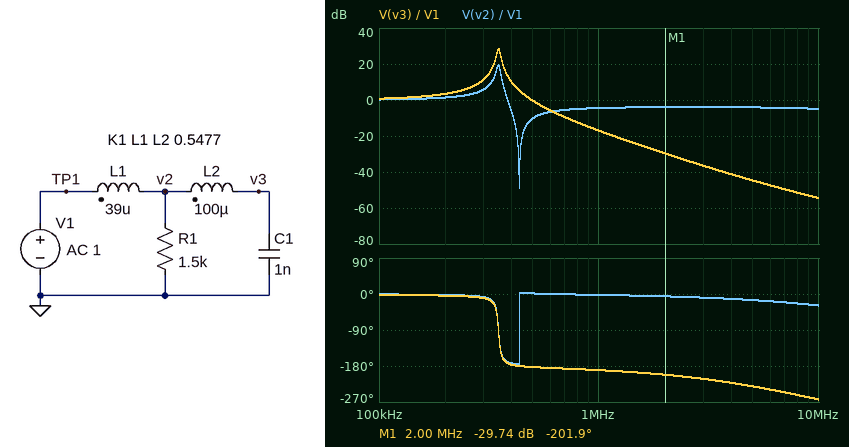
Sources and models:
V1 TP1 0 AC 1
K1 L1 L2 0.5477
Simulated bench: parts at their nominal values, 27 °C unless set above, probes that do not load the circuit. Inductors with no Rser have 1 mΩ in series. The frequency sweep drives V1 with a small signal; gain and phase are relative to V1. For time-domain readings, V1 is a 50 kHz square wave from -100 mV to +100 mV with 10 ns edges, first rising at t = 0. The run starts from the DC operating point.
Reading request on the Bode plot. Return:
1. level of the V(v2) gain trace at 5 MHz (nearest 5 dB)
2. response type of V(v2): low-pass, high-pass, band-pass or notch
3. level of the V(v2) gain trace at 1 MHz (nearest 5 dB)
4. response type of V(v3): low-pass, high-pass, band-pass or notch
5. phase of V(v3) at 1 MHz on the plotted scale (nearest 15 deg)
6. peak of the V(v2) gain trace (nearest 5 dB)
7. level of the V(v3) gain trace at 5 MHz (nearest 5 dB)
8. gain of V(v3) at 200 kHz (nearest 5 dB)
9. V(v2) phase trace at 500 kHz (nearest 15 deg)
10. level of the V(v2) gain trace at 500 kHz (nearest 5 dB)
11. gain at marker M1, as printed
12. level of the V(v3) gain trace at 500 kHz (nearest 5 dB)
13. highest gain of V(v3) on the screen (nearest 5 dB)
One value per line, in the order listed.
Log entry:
-5 dB
band-pass
-5 dB
low-pass
-195 deg
20 dB
-45 dB
5 dB
0 deg
-10 dB
-29.74 dB
0 dB
30 dB
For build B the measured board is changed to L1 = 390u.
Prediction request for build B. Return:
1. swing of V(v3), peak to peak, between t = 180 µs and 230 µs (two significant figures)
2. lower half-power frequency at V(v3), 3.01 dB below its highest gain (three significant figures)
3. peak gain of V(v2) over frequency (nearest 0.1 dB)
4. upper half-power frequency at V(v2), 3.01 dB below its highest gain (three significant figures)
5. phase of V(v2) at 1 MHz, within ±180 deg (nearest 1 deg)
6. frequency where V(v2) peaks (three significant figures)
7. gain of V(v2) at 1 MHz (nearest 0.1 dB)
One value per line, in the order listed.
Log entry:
430 mV
157 kHz
8.3 dB
207 kHz
-6 deg
183 kHz
-11.5 dB
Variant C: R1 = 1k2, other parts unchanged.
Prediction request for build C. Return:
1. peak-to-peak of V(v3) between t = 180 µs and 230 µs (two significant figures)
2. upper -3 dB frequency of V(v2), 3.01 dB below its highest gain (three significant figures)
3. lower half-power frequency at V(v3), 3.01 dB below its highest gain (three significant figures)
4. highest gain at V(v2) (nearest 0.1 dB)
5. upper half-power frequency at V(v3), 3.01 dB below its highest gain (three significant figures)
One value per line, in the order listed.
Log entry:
1.1 V
356 kHz
341 kHz
17.5 dB
358 kHz
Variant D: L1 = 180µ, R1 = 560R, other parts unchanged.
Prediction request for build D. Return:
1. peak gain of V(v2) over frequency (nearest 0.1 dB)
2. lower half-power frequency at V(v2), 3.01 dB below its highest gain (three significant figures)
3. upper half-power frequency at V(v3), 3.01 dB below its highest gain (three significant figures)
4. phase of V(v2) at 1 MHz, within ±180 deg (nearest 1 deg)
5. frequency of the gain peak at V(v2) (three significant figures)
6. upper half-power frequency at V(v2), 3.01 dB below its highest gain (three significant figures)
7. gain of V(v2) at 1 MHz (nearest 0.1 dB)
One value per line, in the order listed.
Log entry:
3.9 dB
108 kHz
285 kHz
-13 deg
222 kHz
265 kHz
-8.9 dB
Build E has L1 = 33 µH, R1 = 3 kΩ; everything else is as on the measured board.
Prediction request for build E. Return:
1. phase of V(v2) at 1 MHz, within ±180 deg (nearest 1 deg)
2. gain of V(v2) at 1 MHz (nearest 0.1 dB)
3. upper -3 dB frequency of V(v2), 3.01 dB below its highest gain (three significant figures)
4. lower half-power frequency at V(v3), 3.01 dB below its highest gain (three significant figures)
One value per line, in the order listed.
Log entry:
-1 deg
-4.1 dB
362 kHz
357 kHz
